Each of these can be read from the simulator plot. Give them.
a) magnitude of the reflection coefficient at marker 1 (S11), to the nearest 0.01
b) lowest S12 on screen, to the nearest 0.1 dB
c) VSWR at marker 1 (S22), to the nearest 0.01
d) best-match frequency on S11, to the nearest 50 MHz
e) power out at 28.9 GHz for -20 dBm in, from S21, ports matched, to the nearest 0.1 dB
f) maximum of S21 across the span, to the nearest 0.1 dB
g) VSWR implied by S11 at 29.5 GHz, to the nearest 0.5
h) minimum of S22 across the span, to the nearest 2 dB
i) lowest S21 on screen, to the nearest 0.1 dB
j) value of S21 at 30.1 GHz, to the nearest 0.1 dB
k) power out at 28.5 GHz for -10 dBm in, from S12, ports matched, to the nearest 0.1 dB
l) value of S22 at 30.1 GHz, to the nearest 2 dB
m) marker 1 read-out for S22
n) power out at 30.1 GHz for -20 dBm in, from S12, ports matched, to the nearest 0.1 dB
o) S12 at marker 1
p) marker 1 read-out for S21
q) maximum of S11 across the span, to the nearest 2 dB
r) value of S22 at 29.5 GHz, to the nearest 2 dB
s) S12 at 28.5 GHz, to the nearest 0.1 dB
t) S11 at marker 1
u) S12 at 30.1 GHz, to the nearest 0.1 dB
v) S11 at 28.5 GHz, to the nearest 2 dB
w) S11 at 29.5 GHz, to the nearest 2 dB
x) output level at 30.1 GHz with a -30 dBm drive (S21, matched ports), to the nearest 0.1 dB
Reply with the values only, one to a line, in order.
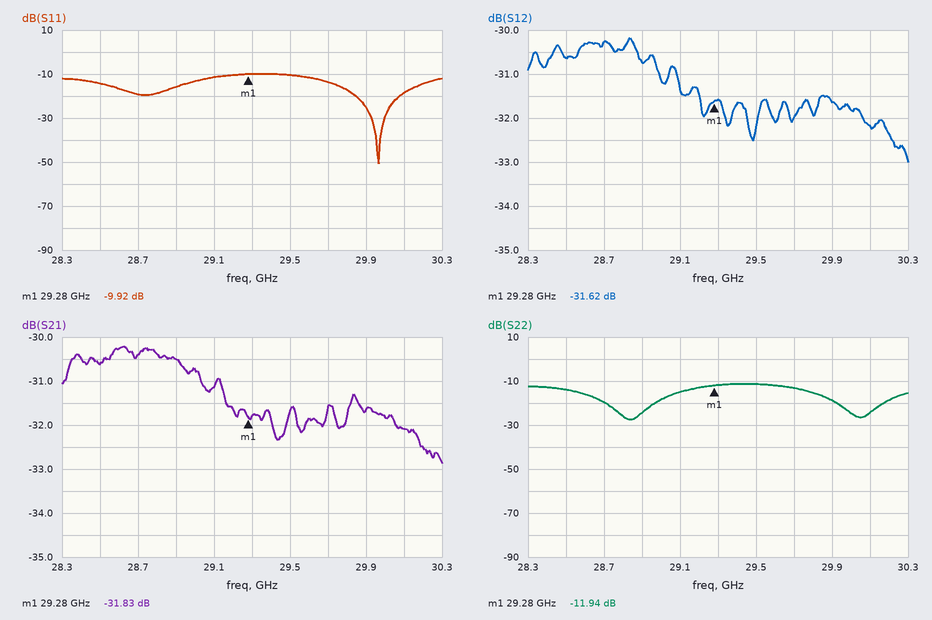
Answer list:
0.32
-33.0 dB
1.68
29.95 GHz
-50.5 dBm
-30.2 dB
2.0
-28 dB
-32.9 dB
-32.1 dB
-40.6 dBm
-24 dB
-11.94 dB
-52.2 dBm
-31.62 dB
-31.83 dB
-10 dB
-12 dB
-30.6 dB
-9.92 dB
-32.2 dB
-14 dB
-10 dB
-62.1 dBm
